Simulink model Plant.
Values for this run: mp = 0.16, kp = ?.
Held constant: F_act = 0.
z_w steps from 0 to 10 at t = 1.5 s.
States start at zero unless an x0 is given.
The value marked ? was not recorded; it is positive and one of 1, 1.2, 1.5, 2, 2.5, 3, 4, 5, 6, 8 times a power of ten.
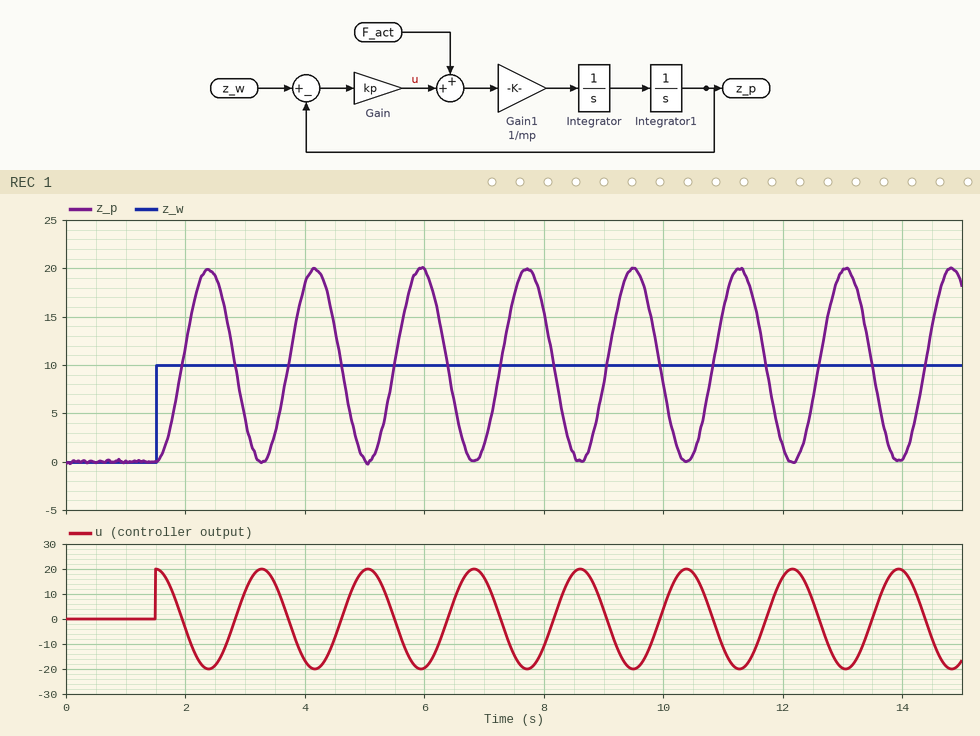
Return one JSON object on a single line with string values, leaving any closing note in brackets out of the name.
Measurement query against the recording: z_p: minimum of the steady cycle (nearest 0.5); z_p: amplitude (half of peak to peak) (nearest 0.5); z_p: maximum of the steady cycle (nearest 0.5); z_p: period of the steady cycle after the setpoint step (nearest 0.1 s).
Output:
{"z_p: minimum of the steady cycle": "0.0", "z_p: amplitude (half of peak to peak)": "10.0", "z_p: maximum of the steady cycle": "20.0", "z_p: period of the steady cycle after the setpoint step": "1.8 s"}
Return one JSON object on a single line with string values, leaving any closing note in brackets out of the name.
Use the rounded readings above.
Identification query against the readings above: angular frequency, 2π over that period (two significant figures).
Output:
{"angular frequency, 2π over that period": "3.5 rad/s"}
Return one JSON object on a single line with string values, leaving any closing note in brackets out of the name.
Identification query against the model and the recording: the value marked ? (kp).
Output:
{"the value marked ?": "2"}
